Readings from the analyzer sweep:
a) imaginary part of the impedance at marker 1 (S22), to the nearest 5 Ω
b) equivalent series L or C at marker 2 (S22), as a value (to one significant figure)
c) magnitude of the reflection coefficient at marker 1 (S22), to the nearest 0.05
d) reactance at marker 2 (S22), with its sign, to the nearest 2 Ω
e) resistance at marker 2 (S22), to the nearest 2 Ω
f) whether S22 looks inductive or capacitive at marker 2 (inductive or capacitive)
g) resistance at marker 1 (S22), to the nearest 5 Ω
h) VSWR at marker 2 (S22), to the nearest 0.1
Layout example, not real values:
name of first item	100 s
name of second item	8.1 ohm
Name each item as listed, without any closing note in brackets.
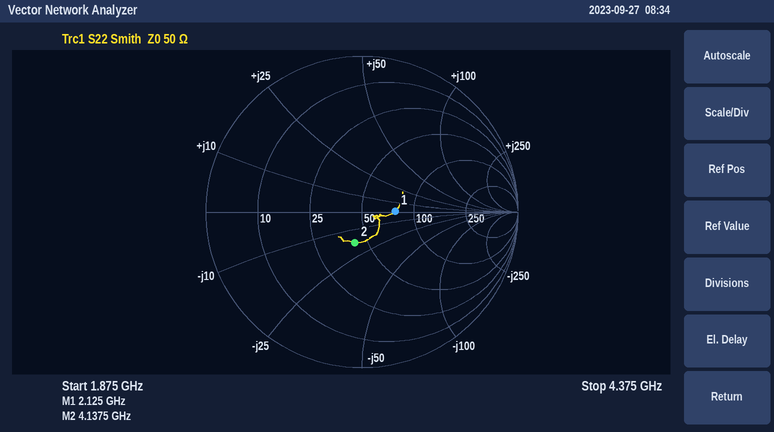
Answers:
imaginary part of the impedance at marker 1 (S22), to the nearest 5 Ω	0 Ω
equivalent series L or C at marker 2 (S22), as a value	2 pF
magnitude of the reflection coefficient at marker 1 (S22), to the nearest 0.05	0.20
reactance at marker 2 (S22), with its sign, to the nearest 2 Ω	-18 Ω
resistance at marker 2 (S22), to the nearest 2 Ω	42 Ω
whether S22 looks inductive or capacitive at marker 2	capacitive
resistance at marker 1 (S22), to the nearest 5 Ω	75 Ω
VSWR at marker 2 (S22), to the nearest 0.1	1.5
